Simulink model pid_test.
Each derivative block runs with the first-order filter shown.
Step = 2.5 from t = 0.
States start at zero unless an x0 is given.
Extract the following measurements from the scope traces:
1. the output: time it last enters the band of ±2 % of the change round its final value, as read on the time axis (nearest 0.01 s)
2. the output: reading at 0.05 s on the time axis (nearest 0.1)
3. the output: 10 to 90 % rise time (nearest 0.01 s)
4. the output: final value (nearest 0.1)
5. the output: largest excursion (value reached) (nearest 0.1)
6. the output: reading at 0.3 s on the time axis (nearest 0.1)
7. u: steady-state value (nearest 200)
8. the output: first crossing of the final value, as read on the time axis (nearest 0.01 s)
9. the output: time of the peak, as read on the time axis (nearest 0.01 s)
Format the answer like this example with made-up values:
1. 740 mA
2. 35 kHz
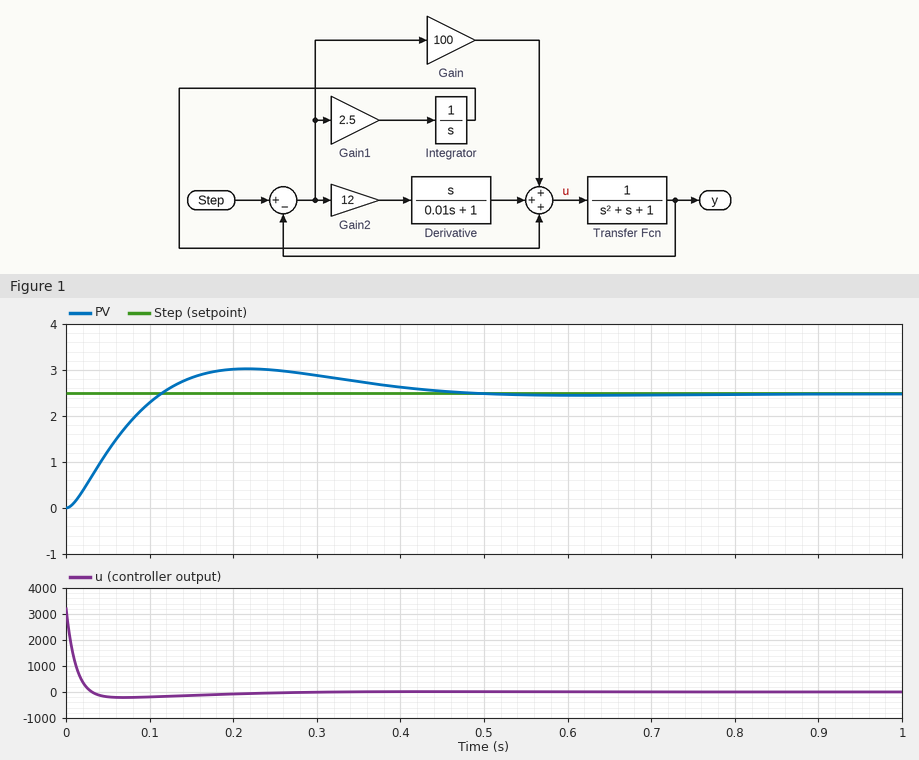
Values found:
1. 0.46 s
2. 1.2
3. 0.08 s
4. 2.5
5. 3.0
6. 2.9
7. 0
8. 0.11 s
9. 0.22 s
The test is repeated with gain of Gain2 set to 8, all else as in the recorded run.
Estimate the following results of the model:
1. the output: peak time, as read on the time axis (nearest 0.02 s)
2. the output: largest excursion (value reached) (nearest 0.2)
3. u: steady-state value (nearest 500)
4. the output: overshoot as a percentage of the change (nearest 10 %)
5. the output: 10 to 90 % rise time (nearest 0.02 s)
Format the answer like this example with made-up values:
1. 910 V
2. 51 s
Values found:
1. 0.24 s
2. 3.2
3. 0
4. 30 %
5. 0.10 s
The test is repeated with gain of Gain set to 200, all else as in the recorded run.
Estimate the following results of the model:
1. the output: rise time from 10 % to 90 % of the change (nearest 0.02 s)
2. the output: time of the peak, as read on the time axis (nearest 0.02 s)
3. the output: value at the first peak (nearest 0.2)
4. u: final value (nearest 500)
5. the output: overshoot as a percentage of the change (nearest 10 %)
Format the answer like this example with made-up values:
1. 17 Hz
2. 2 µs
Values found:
1. 0.06 s
2. 0.16 s
3. 3.4
4. 0
5. 30 %
